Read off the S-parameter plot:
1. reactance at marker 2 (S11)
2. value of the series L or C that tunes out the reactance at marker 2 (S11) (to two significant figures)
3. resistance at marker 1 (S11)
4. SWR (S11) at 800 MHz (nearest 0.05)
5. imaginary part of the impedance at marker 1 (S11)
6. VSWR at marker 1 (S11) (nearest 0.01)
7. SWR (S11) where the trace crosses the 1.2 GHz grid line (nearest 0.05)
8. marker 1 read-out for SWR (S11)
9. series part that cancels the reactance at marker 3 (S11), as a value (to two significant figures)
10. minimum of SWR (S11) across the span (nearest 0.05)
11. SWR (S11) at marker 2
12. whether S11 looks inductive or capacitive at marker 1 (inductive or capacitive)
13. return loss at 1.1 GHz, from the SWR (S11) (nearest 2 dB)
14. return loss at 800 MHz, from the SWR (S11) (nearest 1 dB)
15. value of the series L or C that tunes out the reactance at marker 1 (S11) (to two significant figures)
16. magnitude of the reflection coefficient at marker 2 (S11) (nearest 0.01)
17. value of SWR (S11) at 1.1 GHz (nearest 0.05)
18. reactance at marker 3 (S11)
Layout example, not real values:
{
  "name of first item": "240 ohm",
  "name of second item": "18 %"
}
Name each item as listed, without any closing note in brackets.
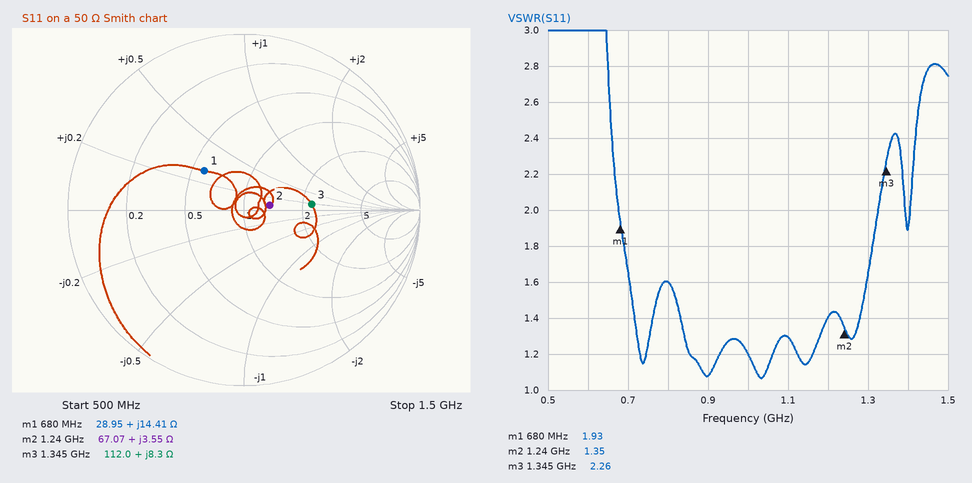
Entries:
{
  "reactance at marker 2": "+3.55 Ω",
  "value of the series L or C that tunes out the reactance at marker 2 (S11)": "36 pF",
  "resistance at marker 1": "28.95 Ω",
  "SWR (S11) at 800 MHz": "1.60",
  "imaginary part of the impedance at marker 1": "+14.41 Ω",
  "VSWR at marker 1 (S11)": "1.93",
  "SWR (S11) where the trace crosses the 1.2 GHz grid line": "1.40",
  "marker 1 read-out for SWR": "1.93",
  "series part that cancels the reactance at marker 3 (S11), as a value": "14 pF",
  "minimum of SWR (S11) across the span": "1.05",
  "SWR (S11) at marker 2": "1.35",
  "whether S11 looks inductive or capacitive at marker 1": "inductive",
  "return loss at 1.1 GHz, from the SWR (S11)": "18 dB",
  "return loss at 800 MHz, from the SWR (S11)": "13 dB",
  "value of the series L or C that tunes out the reactance at marker 1 (S11)": "16 pF",
  "magnitude of the reflection coefficient at marker 2 (S11)": "0.15",
  "value of SWR (S11) at 1.1 GHz": "1.30",
  "reactance at marker 3": "+8.3 Ω"
}
